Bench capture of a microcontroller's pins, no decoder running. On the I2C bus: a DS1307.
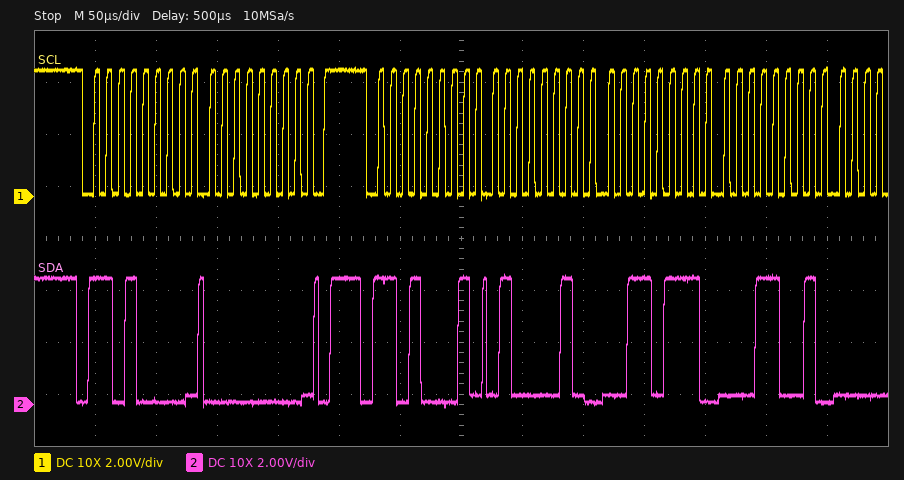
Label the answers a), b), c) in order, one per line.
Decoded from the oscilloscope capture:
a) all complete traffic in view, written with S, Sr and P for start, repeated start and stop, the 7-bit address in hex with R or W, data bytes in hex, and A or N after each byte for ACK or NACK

a) S 68W A 00 A P S 68R A 42 A 37 A 19 A
